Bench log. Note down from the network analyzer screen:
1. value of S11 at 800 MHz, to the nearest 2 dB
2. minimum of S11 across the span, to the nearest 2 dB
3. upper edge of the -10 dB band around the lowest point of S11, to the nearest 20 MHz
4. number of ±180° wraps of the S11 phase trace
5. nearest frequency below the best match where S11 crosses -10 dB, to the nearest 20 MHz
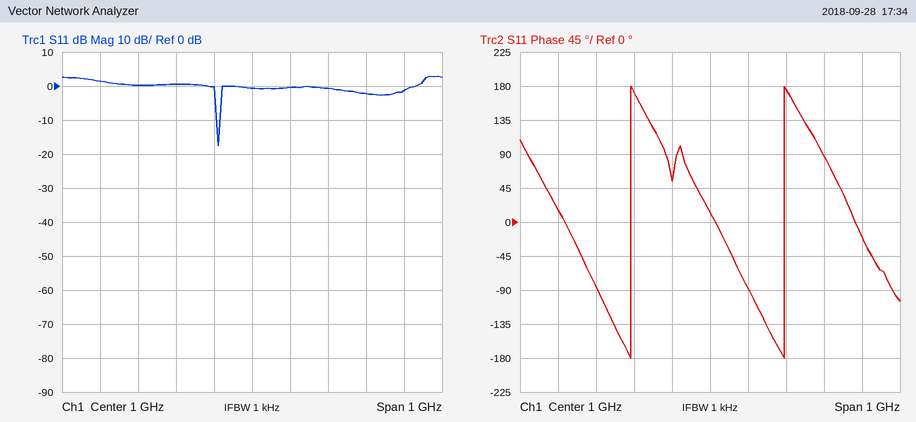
0 dB
-18 dB
920 MHz
2
900 MHz
